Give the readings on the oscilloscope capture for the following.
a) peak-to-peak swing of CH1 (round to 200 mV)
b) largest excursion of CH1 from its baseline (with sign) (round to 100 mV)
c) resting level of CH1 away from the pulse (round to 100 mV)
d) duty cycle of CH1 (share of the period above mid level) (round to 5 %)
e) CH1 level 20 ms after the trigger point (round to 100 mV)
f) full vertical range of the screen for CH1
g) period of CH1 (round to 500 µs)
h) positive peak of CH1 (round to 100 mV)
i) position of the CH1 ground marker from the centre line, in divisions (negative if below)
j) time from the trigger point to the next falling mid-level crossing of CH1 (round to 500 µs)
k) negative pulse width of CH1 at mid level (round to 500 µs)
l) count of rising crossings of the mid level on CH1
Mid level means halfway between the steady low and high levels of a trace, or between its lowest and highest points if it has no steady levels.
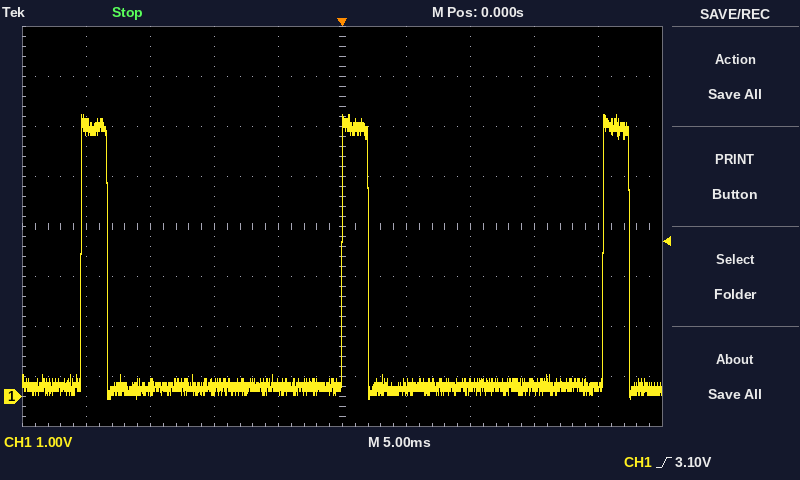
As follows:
5.6 V
+5.4 V
200 mV
10 %
200 mV
8 V
20.5 ms
5.6 V
-3.4 div
2.0 ms
18.5 ms
3
